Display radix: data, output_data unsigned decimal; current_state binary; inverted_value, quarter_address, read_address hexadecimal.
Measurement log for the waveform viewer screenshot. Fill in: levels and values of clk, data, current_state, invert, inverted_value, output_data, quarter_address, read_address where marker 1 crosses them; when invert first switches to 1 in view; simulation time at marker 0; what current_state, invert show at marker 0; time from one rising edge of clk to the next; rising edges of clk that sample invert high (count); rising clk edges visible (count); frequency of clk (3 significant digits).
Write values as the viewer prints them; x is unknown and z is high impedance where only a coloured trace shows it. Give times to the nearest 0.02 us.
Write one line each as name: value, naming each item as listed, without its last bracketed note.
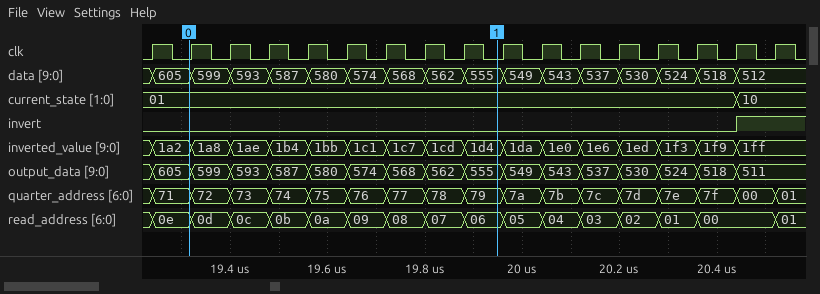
levels and values of clk, data, current_state, invert, inverted_value, output_data, quarter_address, read_address where marker 1 crosses them: clk=0, data=555, current_state=01, invert=0, inverted_value=1d4, output_data=555, quarter_address=79, read_address=06
when invert first switches to 1 in view: 20.44 us
simulation time at marker 0: 19.32 us
what current_state, invert show at marker 0: current_state=01, invert=0
time from one rising edge of clk to the next: 0.08 us
rising edges of clk that sample invert high: 1
rising clk edges visible: 17
frequency of clk: 12.5 MHz
